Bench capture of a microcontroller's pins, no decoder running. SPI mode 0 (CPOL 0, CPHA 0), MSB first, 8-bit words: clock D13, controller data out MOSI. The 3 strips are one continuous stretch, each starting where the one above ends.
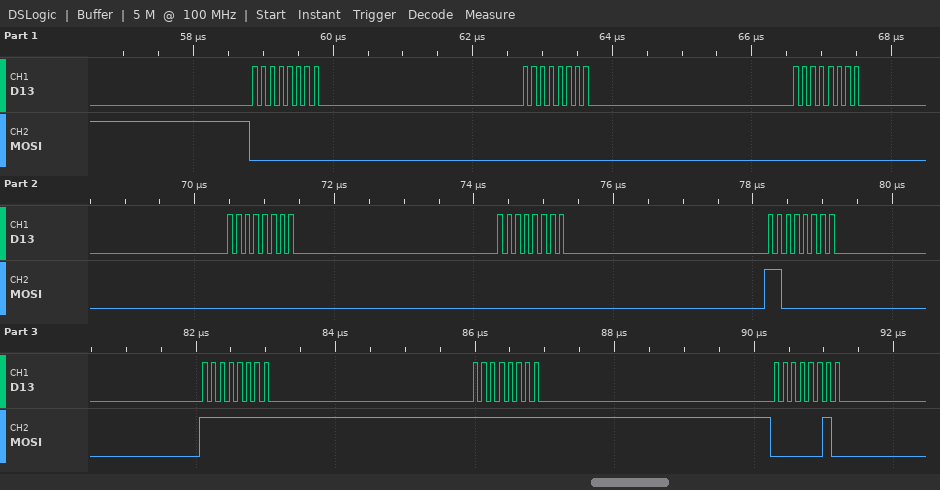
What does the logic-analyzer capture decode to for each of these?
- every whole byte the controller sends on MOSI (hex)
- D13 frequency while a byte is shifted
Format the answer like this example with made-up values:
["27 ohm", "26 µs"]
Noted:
["00 00 00 00 00 C0 FF FF 02", "8 MHz"]
